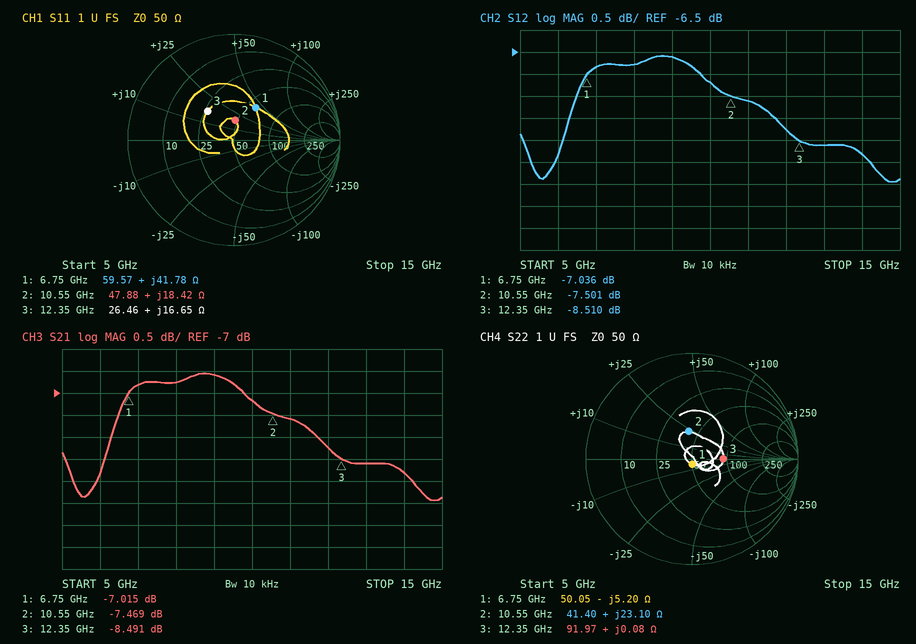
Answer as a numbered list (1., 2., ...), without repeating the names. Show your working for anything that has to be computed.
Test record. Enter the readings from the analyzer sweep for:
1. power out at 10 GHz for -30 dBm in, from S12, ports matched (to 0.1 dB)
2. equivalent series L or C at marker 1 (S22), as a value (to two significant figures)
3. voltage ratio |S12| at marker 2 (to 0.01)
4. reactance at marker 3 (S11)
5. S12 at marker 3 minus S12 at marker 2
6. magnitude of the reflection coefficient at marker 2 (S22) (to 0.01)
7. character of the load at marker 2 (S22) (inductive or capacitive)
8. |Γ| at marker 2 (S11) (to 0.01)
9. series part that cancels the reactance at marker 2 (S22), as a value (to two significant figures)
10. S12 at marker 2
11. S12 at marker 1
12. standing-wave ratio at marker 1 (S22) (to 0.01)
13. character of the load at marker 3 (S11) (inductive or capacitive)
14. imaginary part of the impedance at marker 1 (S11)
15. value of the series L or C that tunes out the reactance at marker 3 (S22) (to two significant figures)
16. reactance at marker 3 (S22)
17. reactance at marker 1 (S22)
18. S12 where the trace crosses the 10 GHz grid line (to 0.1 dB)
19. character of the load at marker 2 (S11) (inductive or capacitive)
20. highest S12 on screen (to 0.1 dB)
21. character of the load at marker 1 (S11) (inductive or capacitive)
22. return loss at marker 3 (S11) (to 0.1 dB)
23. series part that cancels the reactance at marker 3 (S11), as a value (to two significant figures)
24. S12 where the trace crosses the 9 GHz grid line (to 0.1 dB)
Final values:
1. -30 dBm + (-7.2 dB) = -37.2 dBm
2. C = 1/(2π × 6.75 GHz × 5.2 Ω) ≈ 4.5 pF
3. 10^(-7.501/20) ≈ 0.42
4. +16.65 Ω
5. -8.51 − (-7.501) = -1.009 dB
6. 0.26
7. inductive
8. 0.19
9. C = 1/(2π × 10.55 GHz × 23.1 Ω) ≈ 653 fF, so 650 fF to two significant figures
10. -7.501 dB
11. -7.036 dB
12. 1.11
13. inductive
14. +41.78 Ω
15. C = 1/(2π × 12.35 GHz × 0.08 Ω) ≈ 161 pF, so 160 pF to two significant figures
16. +0.08 Ω
17. -5.20 Ω
18. -7.2 dB
19. inductive
20. -6.6 dB
21. inductive
22. 8.7 dB
23. C = 1/(2π × 12.35 GHz × 16.65 Ω) ≈ 774 fF, so 770 fF to two significant figures
24. -6.6 dB
